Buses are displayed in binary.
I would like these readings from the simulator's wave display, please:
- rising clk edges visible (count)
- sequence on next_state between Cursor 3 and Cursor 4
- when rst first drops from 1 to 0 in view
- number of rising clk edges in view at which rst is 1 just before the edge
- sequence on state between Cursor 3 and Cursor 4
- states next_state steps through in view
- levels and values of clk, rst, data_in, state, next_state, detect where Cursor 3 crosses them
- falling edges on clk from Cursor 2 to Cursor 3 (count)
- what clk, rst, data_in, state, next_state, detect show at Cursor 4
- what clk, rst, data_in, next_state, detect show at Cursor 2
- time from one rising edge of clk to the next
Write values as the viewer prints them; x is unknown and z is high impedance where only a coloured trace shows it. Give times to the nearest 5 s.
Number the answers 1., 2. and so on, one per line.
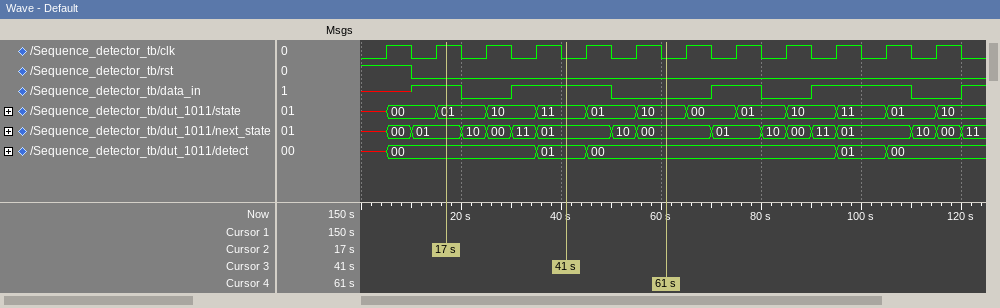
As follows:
1. 12
2. 01, 10, 00
3. 10 s
4. 1
5. 11, 01, 10
6. x, 00, 01, 10, 00, 11, 01, 10, 00, 01, 10, 00, 11, 01, 10, 00, 11
7. clk=0, rst=0, data_in=1, state=11, next_state=01, detect=01
8. 3
9. clk=0, rst=0, data_in=0, state=10, next_state=00, detect=00
10. clk=1, rst=0, data_in=1, next_state=01, detect=00
11. 10 s
